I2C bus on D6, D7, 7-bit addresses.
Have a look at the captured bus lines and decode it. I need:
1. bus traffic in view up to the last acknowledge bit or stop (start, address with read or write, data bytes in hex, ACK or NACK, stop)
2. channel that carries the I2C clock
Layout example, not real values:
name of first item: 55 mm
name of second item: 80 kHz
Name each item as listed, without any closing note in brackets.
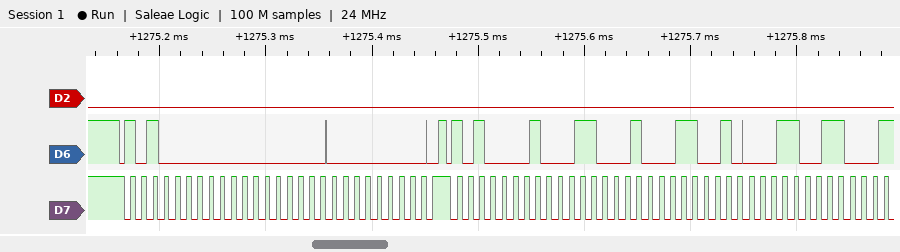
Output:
bus traffic in view up to the last acknowledge bit or stop: start, address 50 write ACK, 00 ACK, 00 ACK, stop, start, address 50 read ACK, 31 ACK, 32 ACK, 33 ACK
channel that carries the I2C clock: D7
